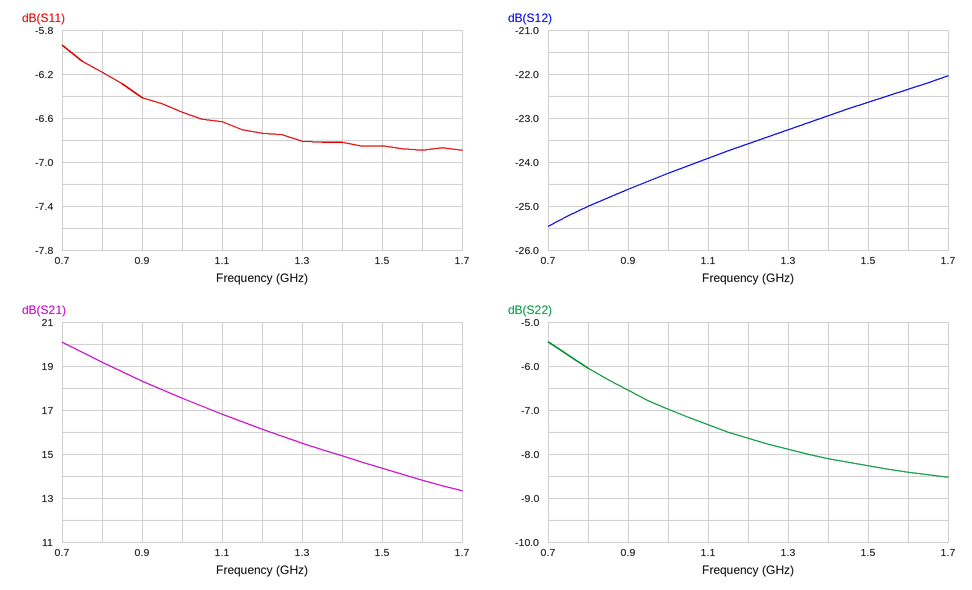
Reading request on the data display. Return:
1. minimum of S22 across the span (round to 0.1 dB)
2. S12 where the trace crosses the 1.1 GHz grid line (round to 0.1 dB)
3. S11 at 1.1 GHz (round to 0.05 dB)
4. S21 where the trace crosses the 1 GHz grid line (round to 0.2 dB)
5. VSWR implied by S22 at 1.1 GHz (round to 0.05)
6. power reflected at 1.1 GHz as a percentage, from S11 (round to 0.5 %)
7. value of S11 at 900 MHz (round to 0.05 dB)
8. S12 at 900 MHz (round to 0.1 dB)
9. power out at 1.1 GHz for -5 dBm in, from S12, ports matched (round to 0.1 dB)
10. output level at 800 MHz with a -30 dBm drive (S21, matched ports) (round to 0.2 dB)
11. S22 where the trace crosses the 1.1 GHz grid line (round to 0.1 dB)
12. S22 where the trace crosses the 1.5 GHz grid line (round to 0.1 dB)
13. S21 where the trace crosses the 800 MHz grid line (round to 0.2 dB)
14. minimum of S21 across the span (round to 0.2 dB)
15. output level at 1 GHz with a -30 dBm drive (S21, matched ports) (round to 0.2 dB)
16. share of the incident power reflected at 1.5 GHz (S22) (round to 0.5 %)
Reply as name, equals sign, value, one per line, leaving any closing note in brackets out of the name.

minimum of S22 across the span = -8.5 dB
S12 where the trace crosses the 1.1 GHz grid line = -23.9 dB
S11 at 1.1 GHz = -6.65 dB
S21 where the trace crosses the 1 GHz grid line = 17.6 dB
VSWR implied by S22 at 1.1 GHz = 2.50
power reflected at 1.1 GHz as a percentage, from S11 = 21.5 %
value of S11 at 900 MHz = -6.40 dB
S12 at 900 MHz = -24.6 dB
power out at 1.1 GHz for -5 dBm in, from S12, ports matched = -28.9 dBm
output level at 800 MHz with a -30 dBm drive (S21, matched ports) = -10.8 dBm
S22 where the trace crosses the 1.1 GHz grid line = -7.3 dB
S22 where the trace crosses the 1.5 GHz grid line = -8.3 dB
S21 where the trace crosses the 800 MHz grid line = 19.2 dB
minimum of S21 across the span = 13.4 dB
output level at 1 GHz with a -30 dBm drive (S21, matched ports) = -12.4 dBm
share of the incident power reflected at 1.5 GHz (S22) = 15.0 %
